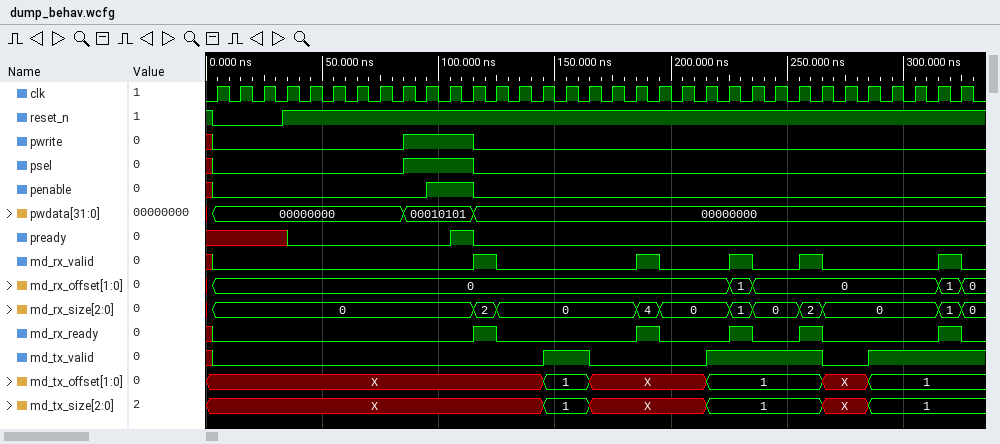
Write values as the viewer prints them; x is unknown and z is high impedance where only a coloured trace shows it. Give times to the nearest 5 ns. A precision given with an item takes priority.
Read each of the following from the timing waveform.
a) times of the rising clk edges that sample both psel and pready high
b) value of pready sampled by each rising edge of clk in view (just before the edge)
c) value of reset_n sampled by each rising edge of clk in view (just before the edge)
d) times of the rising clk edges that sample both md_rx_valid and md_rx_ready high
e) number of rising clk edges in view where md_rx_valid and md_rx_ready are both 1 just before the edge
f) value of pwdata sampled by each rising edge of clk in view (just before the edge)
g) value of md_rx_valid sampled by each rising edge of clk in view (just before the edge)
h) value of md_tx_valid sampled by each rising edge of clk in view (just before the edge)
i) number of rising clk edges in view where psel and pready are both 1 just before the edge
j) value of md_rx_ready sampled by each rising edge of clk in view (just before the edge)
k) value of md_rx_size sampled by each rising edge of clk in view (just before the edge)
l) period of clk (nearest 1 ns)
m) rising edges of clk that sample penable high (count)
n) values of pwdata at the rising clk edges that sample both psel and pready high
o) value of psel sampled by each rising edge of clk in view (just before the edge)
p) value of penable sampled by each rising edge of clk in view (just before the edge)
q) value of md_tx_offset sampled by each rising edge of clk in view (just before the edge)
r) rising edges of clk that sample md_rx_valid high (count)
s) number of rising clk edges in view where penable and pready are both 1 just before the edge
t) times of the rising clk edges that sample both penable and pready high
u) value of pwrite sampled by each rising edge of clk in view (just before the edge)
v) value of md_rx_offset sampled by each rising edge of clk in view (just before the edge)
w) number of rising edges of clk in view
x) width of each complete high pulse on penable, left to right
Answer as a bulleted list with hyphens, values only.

- 115 ns
- x x x x 0 0 0 0 0 0 0 1 0 0 0 0 0 0 0 0 0 0 0 0 0 0 0 0 0 0 0 0 0
- 0 0 0 1 1 1 1 1 1 1 1 1 1 1 1 1 1 1 1 1 1 1 1 1 1 1 1 1 1 1 1 1 1
- 125 ns, 195 ns, 235 ns, 265 ns, 325 ns
- 5
- 00000000, 00000000, 00000000, 00000000, 00000000, 00000000, 00000000, 00000000, 00000000, 00010101, 00010101, 00010101, 00000000, 00000000, 00000000, 00000000, 00000000, 00000000, 00000000, 00000000, 00000000, 00000000, 00000000, 00000000, 00000000, 00000000, 00000000, 00000000, 00000000, 00000000, 00000000, 00000000, 00000000
- 0 0 0 0 0 0 0 0 0 0 0 0 1 0 0 0 0 0 0 1 0 0 0 1 0 0 1 0 0 0 0 0 1
- 0 0 0 0 0 0 0 0 0 0 0 0 0 0 0 1 1 0 0 0 0 0 1 1 1 1 1 0 0 1 1 1 1
- 1
- 0 0 0 0 0 0 0 0 0 0 0 0 1 0 0 0 0 0 0 1 0 0 0 1 0 0 1 0 0 0 0 0 1
- 0, 0, 0, 0, 0, 0, 0, 0, 0, 0, 0, 0, 2, 0, 0, 0, 0, 0, 0, 4, 0, 0, 0, 1, 0, 0, 2, 0, 0, 0, 0, 0, 1
- 10 ns
- 2
- 00010101
- 0 0 0 0 0 0 0 0 0 1 1 1 0 0 0 0 0 0 0 0 0 0 0 0 0 0 0 0 0 0 0 0 0
- 0 0 0 0 0 0 0 0 0 0 1 1 0 0 0 0 0 0 0 0 0 0 0 0 0 0 0 0 0 0 0 0 0
- X, X, X, X, X, X, X, X, X, X, X, X, X, X, X, 1, 1, X, X, X, X, X, 1, 1, 1, 1, 1, X, X, 1, 1, 1, 1
- 5
- 1
- 115 ns
- 0 0 0 0 0 0 0 0 0 1 1 1 0 0 0 0 0 0 0 0 0 0 0 0 0 0 0 0 0 0 0 0 0
- 0, 0, 0, 0, 0, 0, 0, 0, 0, 0, 0, 0, 0, 0, 0, 0, 0, 0, 0, 0, 0, 0, 0, 1, 0, 0, 0, 0, 0, 0, 0, 0, 1
- 33
- 20 ns
